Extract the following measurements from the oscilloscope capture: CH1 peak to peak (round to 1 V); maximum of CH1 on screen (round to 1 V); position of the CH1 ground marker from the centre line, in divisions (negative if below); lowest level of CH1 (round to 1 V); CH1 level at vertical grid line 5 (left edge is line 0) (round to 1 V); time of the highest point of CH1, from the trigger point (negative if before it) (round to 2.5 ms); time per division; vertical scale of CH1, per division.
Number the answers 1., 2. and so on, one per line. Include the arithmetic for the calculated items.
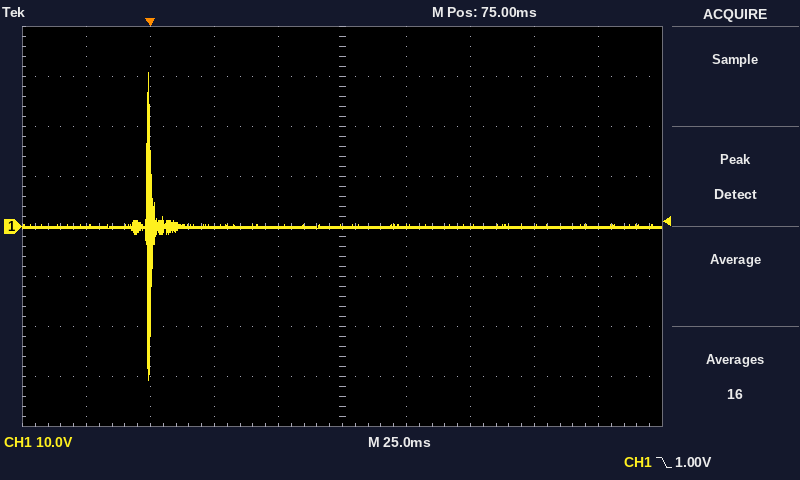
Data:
1. 31 V − (-31 V) = 62 V
2. 31 V
3. 0.0 div
4. -31 V
5. 0 V
6. 0.0 ms
7. 25 ms
8. 10 V
